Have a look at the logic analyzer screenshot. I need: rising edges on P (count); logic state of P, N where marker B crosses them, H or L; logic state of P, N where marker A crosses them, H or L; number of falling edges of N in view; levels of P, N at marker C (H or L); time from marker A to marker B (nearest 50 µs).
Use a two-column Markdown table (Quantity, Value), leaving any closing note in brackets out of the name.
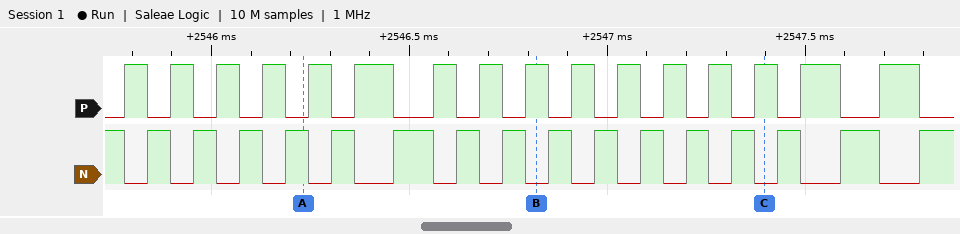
| Quantity | Value |
|---|---|
| rising edges on P | 16 |
| logic state of P, N where marker B crosses them, H or L | P=H, N=L |
| logic state of P, N where marker A crosses them, H or L | P=L, N=H |
| number of falling edges of N in view | 16 |
| levels of P, N at marker C | P=H, N=L |
| time from marker A to marker B | 600 µs |
